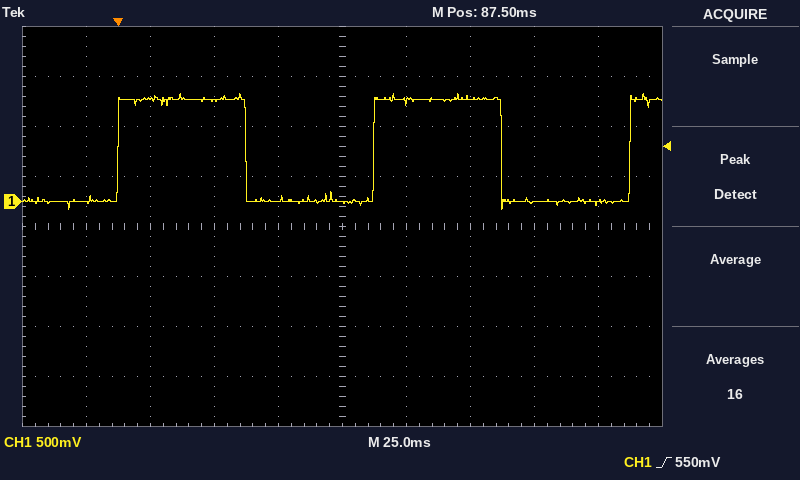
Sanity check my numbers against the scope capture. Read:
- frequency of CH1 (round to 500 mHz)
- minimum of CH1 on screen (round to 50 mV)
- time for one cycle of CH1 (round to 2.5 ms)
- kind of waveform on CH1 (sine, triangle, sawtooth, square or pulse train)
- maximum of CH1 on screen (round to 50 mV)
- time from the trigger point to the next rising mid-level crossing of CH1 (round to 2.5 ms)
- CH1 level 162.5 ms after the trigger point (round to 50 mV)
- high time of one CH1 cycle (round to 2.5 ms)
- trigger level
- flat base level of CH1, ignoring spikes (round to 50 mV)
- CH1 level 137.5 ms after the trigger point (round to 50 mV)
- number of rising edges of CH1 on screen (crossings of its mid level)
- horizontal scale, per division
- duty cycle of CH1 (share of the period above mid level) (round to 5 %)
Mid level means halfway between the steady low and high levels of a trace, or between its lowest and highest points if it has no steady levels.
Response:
10.0 Hz
-100 mV
100.0 ms
square
1.10 V
100.0 ms
0 mV
50.0 ms
550 mV
0 mV
1.05 V
3
25 ms
50 %
